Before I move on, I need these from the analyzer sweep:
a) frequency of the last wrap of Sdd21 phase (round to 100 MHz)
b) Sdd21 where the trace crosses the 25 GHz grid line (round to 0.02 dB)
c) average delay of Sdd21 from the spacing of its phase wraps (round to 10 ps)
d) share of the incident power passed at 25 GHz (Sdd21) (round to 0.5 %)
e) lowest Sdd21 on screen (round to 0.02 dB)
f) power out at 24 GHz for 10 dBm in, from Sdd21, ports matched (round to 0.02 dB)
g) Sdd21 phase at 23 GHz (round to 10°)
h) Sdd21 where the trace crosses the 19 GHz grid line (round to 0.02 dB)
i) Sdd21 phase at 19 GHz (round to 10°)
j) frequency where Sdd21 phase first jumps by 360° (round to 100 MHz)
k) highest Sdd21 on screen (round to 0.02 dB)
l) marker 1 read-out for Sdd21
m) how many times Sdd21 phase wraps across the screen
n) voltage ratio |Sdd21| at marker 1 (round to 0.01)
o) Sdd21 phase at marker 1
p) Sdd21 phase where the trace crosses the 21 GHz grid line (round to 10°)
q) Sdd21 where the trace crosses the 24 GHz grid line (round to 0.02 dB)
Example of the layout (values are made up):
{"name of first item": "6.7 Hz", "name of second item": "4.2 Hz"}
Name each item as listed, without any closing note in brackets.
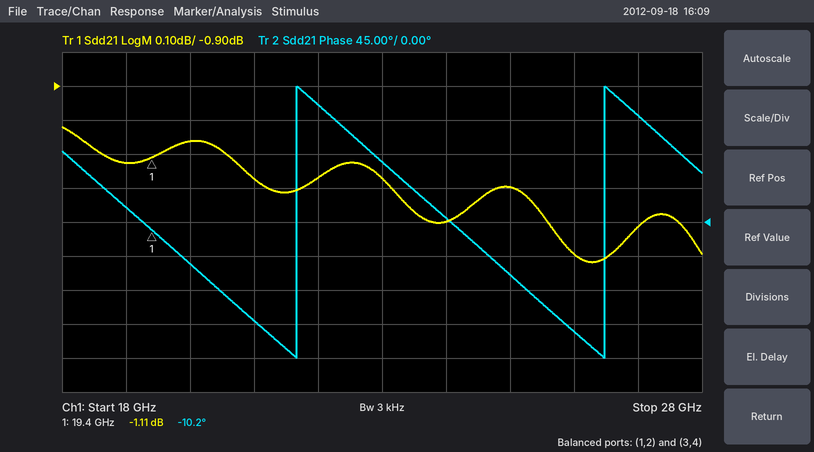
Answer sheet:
{"frequency of the last wrap of Sdd21 phase": "26.5 GHz", "Sdd21 where the trace crosses the 25 GHz grid line": "-1.20 dB", "average delay of Sdd21 from the spacing of its phase wraps": "210 ps", "share of the incident power passed at 25 GHz (Sdd21)": "76.0 %", "lowest Sdd21 on screen": "-1.42 dB", "power out at 24 GHz for 10 dBm in, from Sdd21, ports matched": "8.70 dBm", "Sdd21 phase at 23 GHz": "80°", "Sdd21 where the trace crosses the 19 GHz grid line": "-1.12 dB", "Sdd21 phase at 19 GHz": "20°", "frequency where Sdd21 phase first jumps by 360°": "21.7 GHz", "highest Sdd21 on screen": "-1.02 dB", "marker 1 read-out for Sdd21": "-1.11 dB", "how many times Sdd21 phase wraps across the screen": "2", "voltage ratio |Sdd21| at marker 1": "0.88", "Sdd21 phase at marker 1": "-10.2°", "Sdd21 phase where the trace crosses the 21 GHz grid line": "-130°", "Sdd21 where the trace crosses the 24 GHz grid line": "-1.30 dB"}
